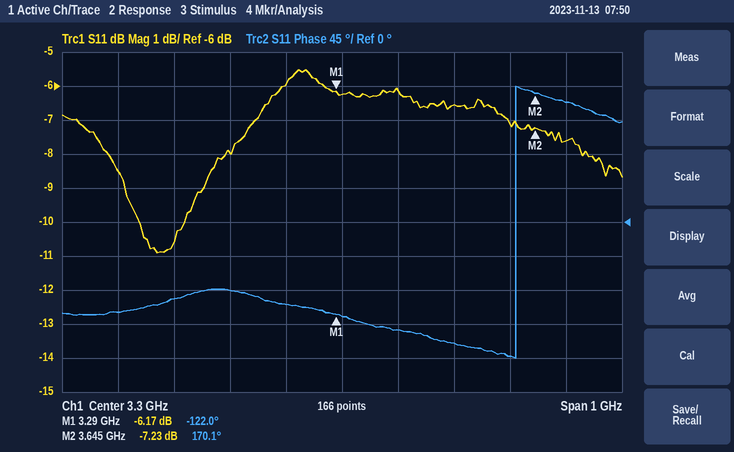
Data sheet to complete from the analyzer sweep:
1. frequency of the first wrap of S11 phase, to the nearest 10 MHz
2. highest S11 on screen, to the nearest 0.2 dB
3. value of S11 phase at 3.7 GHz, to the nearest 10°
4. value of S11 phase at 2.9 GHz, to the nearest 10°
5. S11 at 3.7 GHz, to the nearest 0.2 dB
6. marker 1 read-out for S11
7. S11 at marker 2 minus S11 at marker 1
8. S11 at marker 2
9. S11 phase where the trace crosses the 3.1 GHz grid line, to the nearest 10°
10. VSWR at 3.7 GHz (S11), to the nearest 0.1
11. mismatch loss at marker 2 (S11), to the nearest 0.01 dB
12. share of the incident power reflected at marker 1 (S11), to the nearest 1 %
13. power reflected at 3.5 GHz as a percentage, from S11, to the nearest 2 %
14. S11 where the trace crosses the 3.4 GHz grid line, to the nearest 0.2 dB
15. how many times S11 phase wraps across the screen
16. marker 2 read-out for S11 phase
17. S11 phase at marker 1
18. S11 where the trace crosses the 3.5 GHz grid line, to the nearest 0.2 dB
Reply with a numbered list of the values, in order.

1. 3.61 GHz
2. -5.6 dB
3. 160°
4. -120°
5. -7.6 dB
6. -6.17 dB
7. -1.06 dB
8. -7.23 dB
9. -90°
10. 2.4
11. 0.91 dB
12. 24 %
13. 22 %
14. -6.2 dB
15. 1
16. 170.1°
17. -122.0°
18. -6.6 dB
